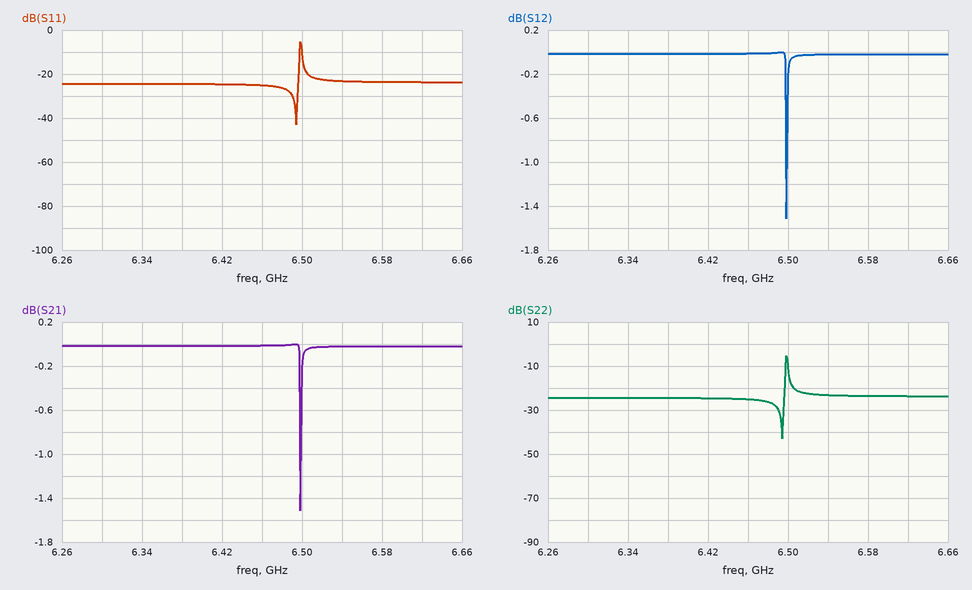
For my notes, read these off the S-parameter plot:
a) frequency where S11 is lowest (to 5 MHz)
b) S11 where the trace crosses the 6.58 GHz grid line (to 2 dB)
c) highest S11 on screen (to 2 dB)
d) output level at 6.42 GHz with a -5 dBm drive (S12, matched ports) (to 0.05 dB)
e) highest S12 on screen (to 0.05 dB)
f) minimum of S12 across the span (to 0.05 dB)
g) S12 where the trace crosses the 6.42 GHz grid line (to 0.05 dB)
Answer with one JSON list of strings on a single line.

["6.495 GHz", "-24 dB", "-6 dB", "-5.00 dBm", "0.00 dB", "-1.50 dB", "0.00 dB"]
